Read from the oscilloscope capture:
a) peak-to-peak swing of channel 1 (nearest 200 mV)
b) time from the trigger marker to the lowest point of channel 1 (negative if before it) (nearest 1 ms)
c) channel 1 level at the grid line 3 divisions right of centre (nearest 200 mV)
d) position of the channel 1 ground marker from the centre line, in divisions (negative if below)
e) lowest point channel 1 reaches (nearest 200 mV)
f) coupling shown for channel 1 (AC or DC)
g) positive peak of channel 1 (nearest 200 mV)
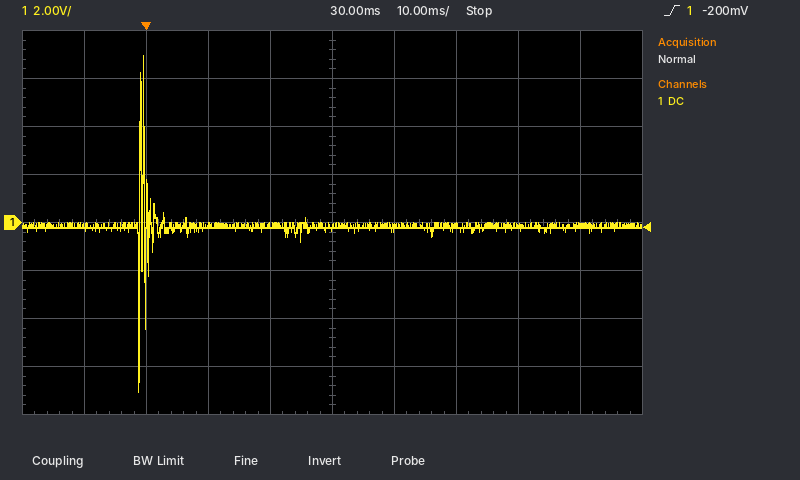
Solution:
14.0 V
-1 ms
-200 mV
0.0 div
-7.0 V
DC
7.0 V
